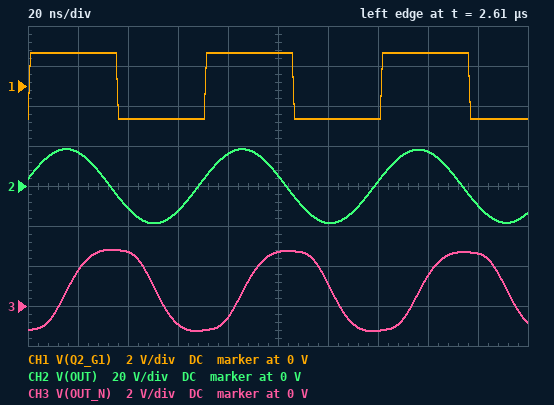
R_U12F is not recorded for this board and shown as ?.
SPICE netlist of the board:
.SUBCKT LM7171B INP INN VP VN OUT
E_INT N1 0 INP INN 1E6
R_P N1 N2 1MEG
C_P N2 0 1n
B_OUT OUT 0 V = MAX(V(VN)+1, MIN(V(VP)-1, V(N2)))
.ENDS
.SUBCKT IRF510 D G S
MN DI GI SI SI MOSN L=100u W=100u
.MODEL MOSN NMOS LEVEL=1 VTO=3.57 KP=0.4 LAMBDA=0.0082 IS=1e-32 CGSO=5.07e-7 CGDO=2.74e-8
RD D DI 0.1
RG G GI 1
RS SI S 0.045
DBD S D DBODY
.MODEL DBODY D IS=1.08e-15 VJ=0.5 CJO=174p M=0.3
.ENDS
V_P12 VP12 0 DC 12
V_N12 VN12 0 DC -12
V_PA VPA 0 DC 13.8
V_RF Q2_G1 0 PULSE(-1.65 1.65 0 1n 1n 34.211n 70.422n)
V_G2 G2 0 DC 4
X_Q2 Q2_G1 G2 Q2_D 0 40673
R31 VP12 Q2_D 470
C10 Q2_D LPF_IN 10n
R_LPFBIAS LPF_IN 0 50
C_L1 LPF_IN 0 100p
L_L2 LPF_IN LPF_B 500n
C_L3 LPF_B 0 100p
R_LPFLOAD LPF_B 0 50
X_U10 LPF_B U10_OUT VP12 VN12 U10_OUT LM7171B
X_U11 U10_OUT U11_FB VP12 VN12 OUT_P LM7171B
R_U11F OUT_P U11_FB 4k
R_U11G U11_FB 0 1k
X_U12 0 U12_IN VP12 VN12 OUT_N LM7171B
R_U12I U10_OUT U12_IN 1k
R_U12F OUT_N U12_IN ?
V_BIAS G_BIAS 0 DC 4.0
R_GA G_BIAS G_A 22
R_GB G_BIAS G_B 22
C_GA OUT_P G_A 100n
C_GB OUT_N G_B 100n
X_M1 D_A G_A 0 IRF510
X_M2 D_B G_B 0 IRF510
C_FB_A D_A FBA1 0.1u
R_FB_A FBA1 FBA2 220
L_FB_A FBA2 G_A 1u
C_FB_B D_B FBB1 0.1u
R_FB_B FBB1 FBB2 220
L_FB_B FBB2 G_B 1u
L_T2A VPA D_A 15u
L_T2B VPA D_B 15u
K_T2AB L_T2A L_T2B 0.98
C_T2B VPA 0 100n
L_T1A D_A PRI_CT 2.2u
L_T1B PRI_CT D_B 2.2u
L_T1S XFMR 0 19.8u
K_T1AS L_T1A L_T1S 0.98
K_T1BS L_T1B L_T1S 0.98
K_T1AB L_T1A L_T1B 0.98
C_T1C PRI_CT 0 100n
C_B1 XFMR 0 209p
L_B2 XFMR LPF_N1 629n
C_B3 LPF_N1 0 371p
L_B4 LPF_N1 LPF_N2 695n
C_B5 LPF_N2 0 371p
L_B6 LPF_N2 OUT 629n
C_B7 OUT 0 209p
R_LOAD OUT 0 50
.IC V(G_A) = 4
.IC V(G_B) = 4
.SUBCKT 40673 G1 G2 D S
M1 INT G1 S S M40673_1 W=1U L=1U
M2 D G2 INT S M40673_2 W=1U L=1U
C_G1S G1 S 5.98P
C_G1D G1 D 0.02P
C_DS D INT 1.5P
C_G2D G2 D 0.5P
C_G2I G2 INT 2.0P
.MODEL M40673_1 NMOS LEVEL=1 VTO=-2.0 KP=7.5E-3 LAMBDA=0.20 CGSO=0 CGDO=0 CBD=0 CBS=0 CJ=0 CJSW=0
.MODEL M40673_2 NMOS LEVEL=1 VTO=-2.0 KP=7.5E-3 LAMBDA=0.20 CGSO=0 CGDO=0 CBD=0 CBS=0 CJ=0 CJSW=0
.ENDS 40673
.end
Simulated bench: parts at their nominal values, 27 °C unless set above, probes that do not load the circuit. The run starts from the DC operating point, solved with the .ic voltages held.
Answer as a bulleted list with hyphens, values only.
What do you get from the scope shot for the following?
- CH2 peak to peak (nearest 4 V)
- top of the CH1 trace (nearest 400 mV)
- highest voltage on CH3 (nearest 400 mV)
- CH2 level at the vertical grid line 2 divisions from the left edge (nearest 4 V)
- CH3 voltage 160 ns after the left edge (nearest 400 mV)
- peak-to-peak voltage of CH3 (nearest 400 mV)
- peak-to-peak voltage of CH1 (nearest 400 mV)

- 36 V
- 1.6 V
- 2.8 V
- -12 V
- 1.6 V
- 4.0 V
- 3.2 V
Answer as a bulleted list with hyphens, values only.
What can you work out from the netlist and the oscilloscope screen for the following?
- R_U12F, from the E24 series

- 3 kΩ
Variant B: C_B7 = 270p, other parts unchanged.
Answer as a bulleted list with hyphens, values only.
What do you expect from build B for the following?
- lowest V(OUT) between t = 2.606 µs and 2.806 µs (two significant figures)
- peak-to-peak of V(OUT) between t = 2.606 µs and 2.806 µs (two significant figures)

- -18 V
- 35 V
